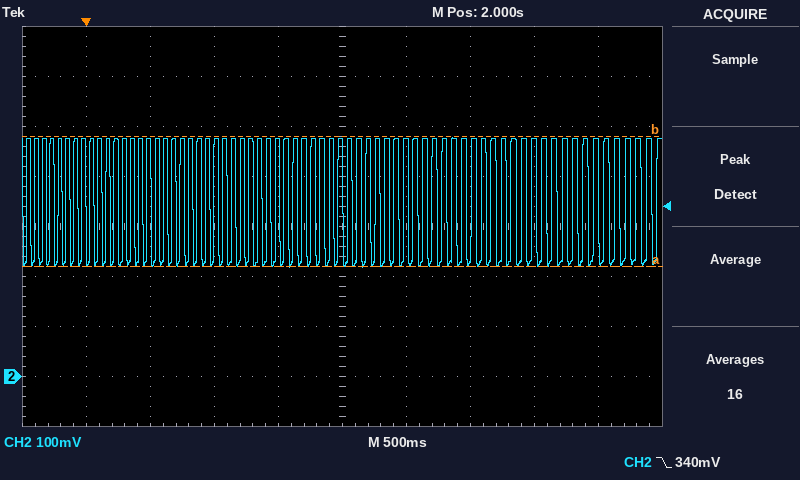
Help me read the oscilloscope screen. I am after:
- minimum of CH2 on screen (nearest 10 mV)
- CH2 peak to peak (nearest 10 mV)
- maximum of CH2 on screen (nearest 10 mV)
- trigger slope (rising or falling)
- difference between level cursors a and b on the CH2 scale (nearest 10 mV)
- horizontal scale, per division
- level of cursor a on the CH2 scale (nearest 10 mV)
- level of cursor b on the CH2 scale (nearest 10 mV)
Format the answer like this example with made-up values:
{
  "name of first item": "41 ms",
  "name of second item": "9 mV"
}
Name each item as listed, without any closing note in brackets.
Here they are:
{
  "minimum of CH2 on screen": "220 mV",
  "CH2 peak to peak": "260 mV",
  "maximum of CH2 on screen": "480 mV",
  "trigger slope": "falling",
  "difference between level cursors a and b on the CH2 scale": "260 mV",
  "horizontal scale, per division": "500 ms",
  "level of cursor a on the CH2 scale": "220 mV",
  "level of cursor b on the CH2 scale": "480 mV"
}
